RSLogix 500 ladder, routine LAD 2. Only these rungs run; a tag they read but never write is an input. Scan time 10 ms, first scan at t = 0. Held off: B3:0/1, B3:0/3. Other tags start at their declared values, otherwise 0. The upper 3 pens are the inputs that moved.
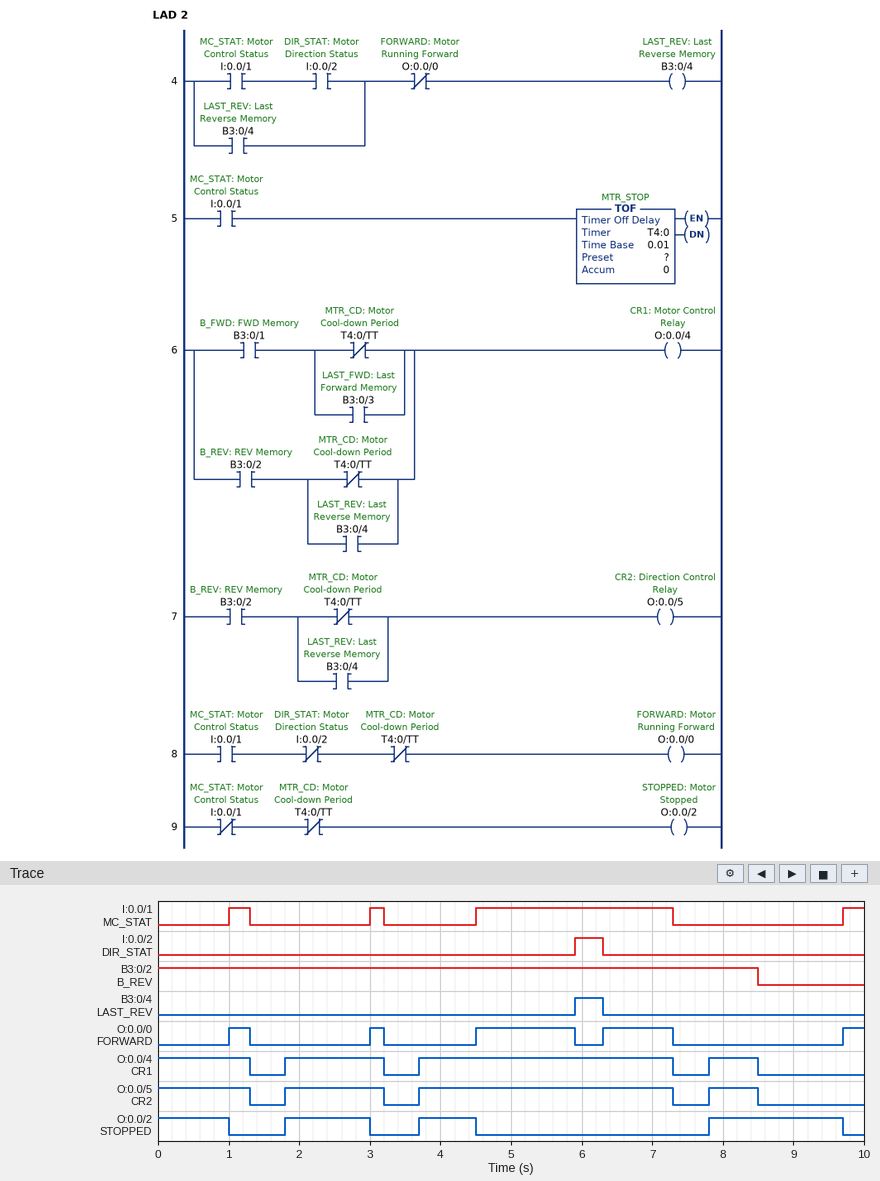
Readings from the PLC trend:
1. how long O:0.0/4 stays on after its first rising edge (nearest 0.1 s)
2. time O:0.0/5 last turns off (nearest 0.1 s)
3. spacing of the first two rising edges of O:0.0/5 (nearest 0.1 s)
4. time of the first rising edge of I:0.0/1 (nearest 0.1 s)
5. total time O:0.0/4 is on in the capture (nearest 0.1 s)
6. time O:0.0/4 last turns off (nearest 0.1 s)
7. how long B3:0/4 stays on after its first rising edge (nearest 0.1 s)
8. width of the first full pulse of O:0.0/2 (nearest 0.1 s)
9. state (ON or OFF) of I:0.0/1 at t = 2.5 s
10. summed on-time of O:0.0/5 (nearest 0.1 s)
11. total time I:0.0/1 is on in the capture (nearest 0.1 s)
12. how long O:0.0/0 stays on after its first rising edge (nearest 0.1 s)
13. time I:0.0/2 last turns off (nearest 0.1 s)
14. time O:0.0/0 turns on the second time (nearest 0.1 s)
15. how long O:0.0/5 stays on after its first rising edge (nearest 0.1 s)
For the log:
1.4 s
8.5 s
1.9 s
1.0 s
7.0 s
8.5 s
0.4 s
1.2 s
OFF
7.0 s
3.6 s
0.3 s
6.3 s
3.0 s
1.4 s
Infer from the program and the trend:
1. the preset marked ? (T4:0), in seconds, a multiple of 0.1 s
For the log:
0.5 s
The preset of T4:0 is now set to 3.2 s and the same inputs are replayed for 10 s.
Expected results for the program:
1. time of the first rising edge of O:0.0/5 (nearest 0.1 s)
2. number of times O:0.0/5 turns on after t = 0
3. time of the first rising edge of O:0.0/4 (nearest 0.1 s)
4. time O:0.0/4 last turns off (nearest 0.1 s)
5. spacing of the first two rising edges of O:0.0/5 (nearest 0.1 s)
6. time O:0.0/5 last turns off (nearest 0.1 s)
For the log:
3.0 s
2
3.0 s
7.3 s
1.5 s
7.3 s
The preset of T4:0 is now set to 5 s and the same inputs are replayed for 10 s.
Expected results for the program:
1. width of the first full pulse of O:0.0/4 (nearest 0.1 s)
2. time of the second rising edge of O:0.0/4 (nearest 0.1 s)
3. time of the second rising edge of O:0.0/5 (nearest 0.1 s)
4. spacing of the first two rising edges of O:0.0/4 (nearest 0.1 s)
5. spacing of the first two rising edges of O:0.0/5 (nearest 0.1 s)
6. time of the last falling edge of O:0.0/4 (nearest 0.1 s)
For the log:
0.2 s
4.5 s
4.5 s
1.5 s
1.5 s
7.3 s
